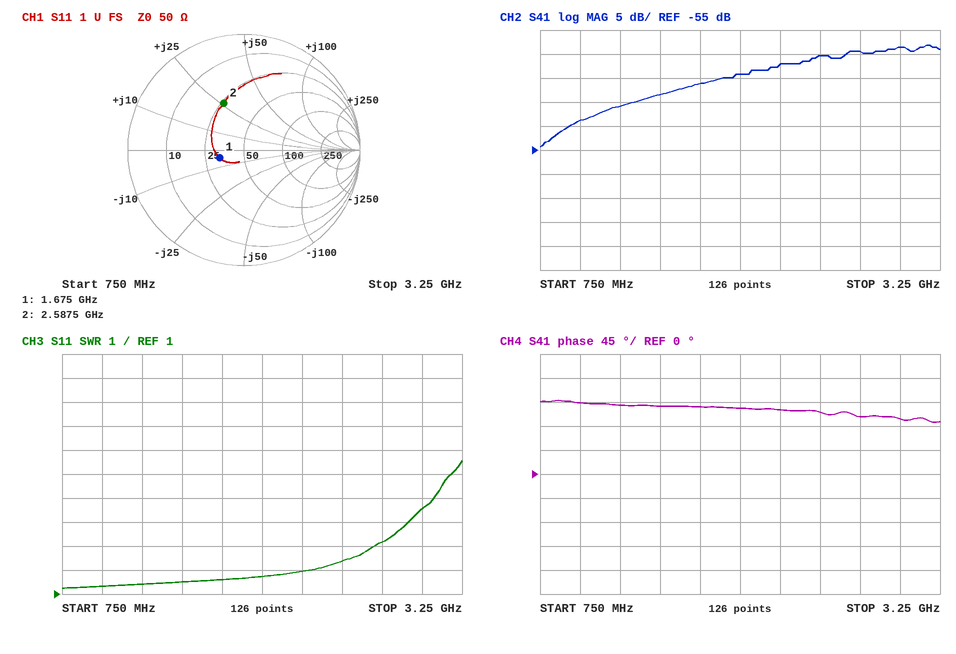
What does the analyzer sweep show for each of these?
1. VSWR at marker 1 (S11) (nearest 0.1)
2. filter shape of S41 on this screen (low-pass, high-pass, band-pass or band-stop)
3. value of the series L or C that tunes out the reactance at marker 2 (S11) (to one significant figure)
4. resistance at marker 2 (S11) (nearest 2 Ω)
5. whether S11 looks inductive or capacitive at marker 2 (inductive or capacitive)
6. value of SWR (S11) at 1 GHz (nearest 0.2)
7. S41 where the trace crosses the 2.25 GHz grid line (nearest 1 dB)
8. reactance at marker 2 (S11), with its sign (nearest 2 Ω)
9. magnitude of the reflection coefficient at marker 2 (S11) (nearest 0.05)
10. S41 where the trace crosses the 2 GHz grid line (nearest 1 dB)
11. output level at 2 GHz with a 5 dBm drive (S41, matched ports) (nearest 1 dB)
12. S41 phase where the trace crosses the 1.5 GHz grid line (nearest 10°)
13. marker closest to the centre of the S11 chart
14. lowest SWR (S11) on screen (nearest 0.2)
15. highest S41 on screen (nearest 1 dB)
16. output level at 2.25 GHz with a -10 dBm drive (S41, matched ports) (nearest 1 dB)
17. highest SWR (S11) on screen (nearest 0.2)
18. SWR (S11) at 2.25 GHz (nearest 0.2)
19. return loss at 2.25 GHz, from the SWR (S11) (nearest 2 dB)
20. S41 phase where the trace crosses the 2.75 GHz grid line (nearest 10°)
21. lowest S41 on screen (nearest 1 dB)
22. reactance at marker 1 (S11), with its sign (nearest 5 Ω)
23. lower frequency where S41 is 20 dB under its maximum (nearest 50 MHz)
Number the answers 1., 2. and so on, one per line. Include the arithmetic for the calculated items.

1. 1.6
2. high-pass
3. C = 1/(2π × 2.5875 GHz × 26 Ω) ≈ 2 pF
4. 26 Ω
5. inductive
6. 1.4
7. -37 dB
8. +26 Ω
9. 0.45
10. -39 dB
11. 5 dBm + (-39 dB) = -34 dBm
12. 130°
13. marker 1
14. 1.2
15. -33 dB
16. -10 dBm + (-37 dB) = -47 dBm
17. 6.6
18. 2.0
19. −20 log10((2 − 1)/(2 + 1)) ≈ 10 dB
20. 110°
21. -54 dB
22. -5 Ω
23. 800 MHz
